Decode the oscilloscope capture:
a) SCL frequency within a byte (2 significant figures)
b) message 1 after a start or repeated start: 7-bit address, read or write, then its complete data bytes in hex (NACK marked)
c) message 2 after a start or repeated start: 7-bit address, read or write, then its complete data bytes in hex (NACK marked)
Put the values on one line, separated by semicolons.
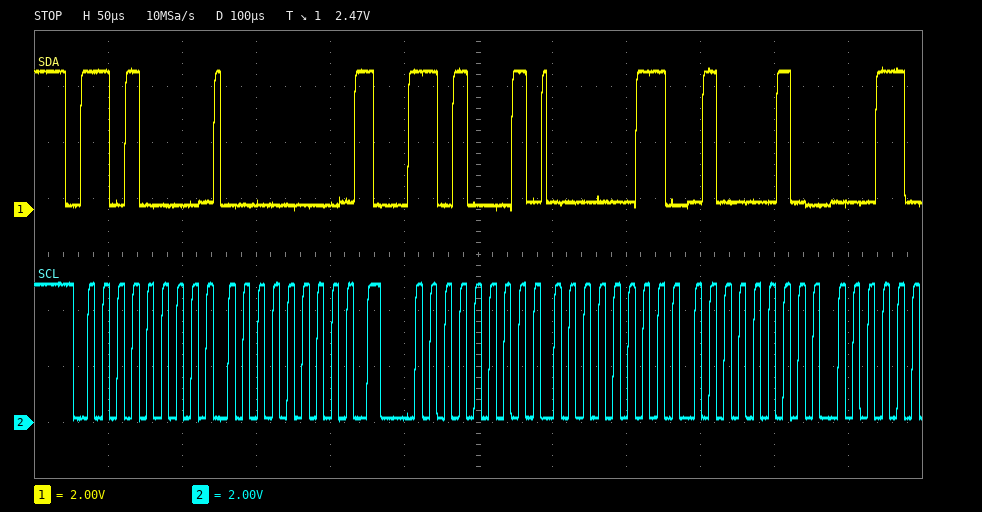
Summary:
100 kHz; 0x68 write: 00; 0x68 read: 03 42
